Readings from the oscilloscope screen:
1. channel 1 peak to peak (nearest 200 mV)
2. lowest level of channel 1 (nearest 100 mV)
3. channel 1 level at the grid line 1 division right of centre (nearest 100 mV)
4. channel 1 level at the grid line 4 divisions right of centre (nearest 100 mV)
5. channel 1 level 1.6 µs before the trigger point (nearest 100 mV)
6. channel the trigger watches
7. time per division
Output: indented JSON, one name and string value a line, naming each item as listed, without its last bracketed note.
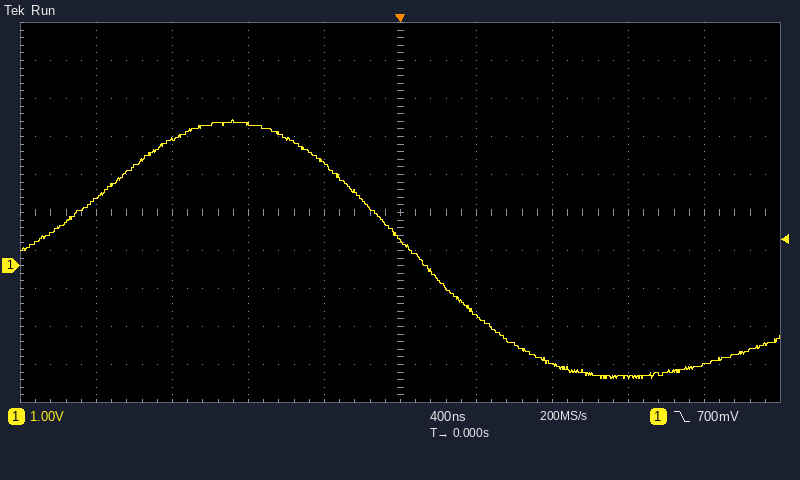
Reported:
{
  "channel 1 peak to peak": "6.8 V",
  "lowest level of channel 1": "-3.0 V",
  "channel 1 level at the grid line 1 division right of centre": "-1.3 V",
  "channel 1 level at the grid line 4 divisions right of centre": "-2.6 V",
  "channel 1 level 1.6 µs before the trigger point": "1.8 V",
  "channel the trigger watches": "channel 1",
  "time per division": "400 ns"
}
